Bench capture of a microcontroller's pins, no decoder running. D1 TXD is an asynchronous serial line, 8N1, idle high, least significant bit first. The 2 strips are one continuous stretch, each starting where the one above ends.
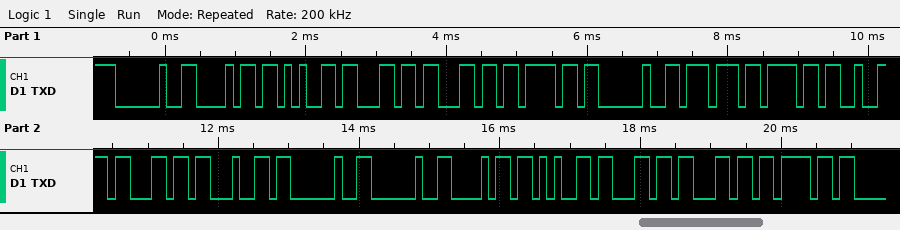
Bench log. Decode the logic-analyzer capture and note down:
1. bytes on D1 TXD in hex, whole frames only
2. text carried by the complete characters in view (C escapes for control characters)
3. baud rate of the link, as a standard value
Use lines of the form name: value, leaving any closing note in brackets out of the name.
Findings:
bytes on D1 TXD in hex, whole frames only: 0x20 0x68 0x65 0x6C 0x6C 0x6F 0x20 0x77 0x6F 0x72 0x6C 0x64 0x20 0x20 0x68 0x65 0x6C 0x6C 0x6F
text carried by the complete characters in view: " hello world  hello"
baud rate of the link, as a standard value: 9600 baud
